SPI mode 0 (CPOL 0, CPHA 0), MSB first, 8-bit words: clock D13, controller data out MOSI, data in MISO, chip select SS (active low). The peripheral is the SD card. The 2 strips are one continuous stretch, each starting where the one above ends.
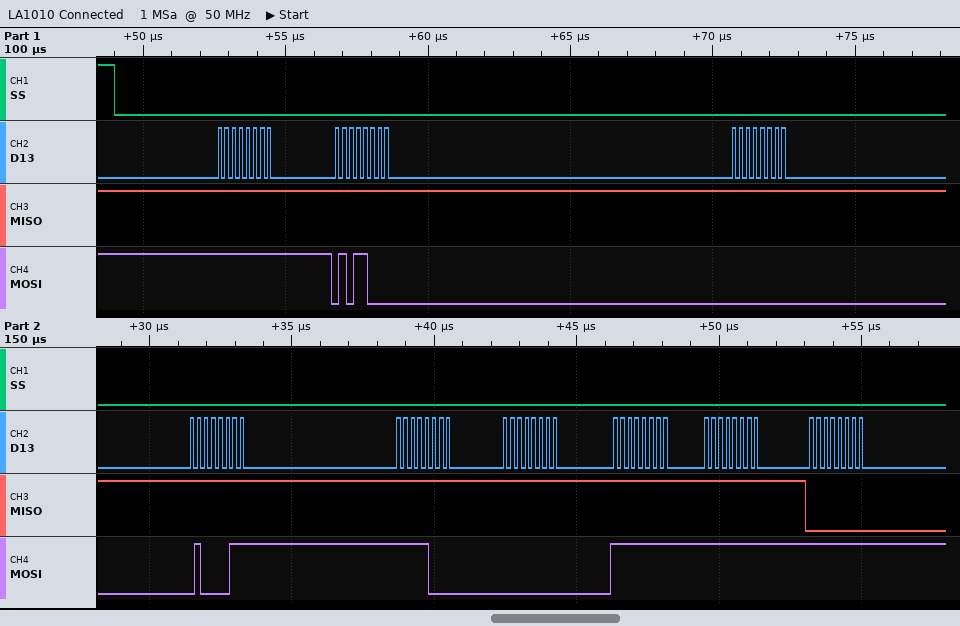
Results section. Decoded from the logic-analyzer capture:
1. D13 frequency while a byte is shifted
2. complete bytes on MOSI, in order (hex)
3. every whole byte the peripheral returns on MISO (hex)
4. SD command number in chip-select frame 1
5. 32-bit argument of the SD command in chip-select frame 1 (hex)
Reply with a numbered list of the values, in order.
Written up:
1. 4 MHz
2. FF 58 00 43 F8 00 FF FF FF
3. FF FF FF FF FF FF FF FF 00
4. CMD24
5. 0x0043F800
